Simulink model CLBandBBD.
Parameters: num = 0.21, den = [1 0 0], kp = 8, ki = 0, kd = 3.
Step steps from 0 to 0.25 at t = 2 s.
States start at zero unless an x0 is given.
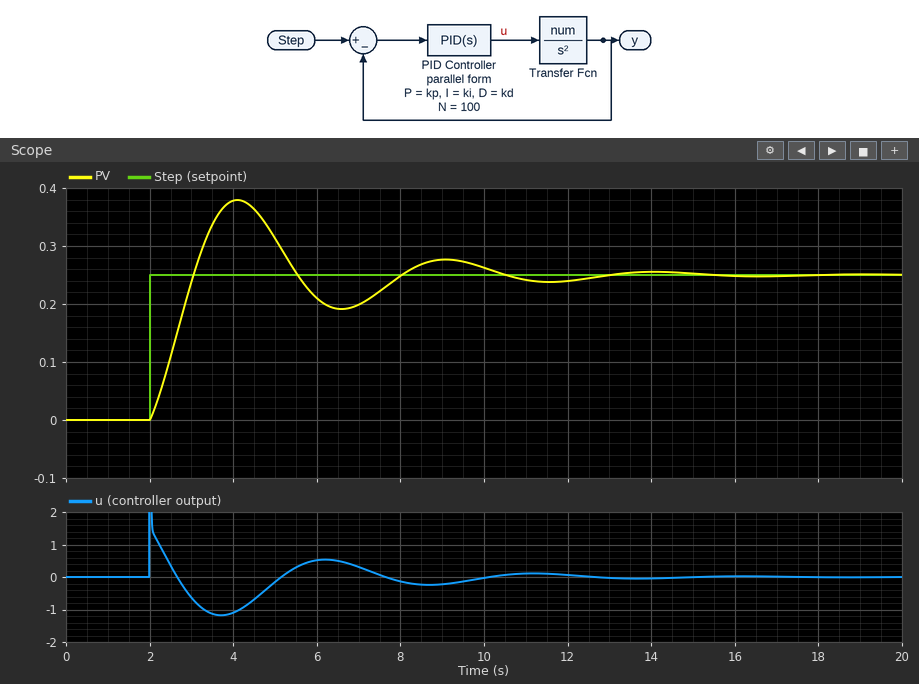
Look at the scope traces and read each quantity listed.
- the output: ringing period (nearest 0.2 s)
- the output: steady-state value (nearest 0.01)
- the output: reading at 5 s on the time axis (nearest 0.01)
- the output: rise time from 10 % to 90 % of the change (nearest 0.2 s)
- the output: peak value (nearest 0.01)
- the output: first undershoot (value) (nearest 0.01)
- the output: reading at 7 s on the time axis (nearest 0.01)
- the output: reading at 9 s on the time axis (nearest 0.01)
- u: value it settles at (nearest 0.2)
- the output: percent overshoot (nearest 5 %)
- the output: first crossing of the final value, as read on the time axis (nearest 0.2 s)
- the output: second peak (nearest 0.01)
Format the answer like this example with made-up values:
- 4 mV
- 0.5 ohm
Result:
- 5.0 s
- 0.25
- 0.31
- 0.8 s
- 0.38
- 0.19
- 0.20
- 0.28
- 0.0
- 50 %
- 3.0 s
- 0.28
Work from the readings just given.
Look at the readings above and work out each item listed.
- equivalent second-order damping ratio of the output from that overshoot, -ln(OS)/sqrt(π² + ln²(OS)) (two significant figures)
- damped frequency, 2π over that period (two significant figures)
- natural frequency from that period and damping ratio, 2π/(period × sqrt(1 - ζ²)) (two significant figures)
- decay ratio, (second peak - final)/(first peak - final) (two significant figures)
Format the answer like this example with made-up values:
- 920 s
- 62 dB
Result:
- 0.22
- 1.3 rad/s
- 1.3 rad/s
- 0.23
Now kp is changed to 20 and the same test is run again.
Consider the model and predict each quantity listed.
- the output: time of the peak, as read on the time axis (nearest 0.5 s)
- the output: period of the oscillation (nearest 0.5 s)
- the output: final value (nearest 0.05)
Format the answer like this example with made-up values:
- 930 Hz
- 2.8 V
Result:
- 3.5 s
- 3.0 s
- 0.25
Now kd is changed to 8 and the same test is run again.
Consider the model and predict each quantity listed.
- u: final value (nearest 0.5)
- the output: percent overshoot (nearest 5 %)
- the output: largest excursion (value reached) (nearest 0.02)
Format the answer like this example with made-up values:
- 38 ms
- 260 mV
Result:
- 0.0
- 25 %
- 0.30
